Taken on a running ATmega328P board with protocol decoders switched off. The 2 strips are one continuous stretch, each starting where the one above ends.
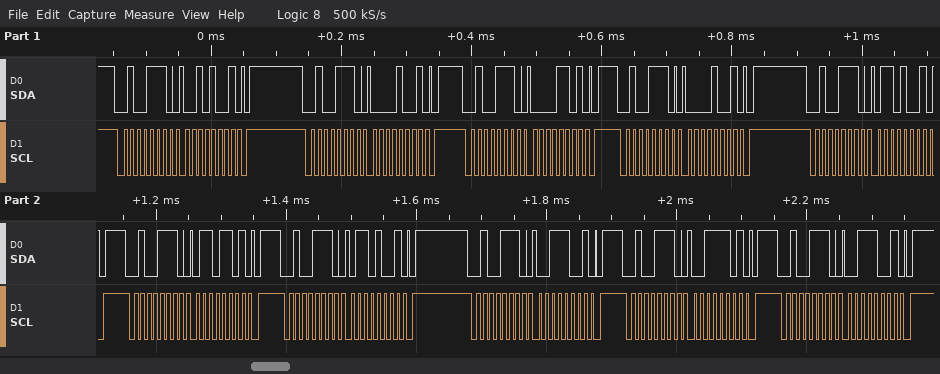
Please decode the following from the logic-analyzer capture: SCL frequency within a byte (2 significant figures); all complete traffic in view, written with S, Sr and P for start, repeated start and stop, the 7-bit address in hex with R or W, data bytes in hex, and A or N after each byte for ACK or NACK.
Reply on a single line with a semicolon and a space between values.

100 kHz; S 27W A 29 A P S 27W A 09 A P S 27W A 0D A P S 27W A 09 A P S 27W A 69 A P S 27W A 6D A P S 27W A 69 A P S 27W A 39 A P S 27W A 3D A P S 27W A 39 A P
